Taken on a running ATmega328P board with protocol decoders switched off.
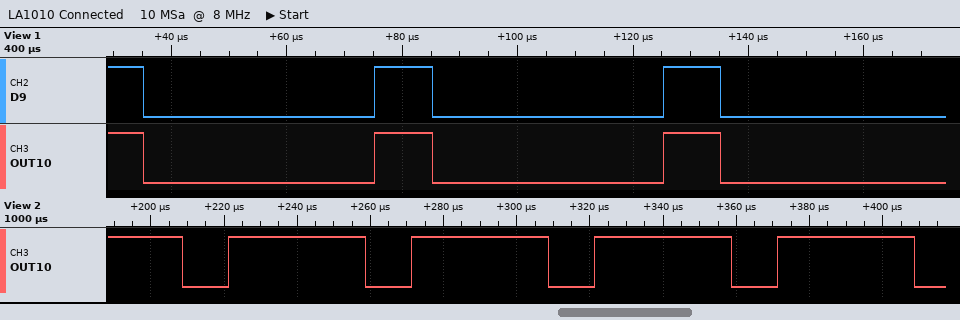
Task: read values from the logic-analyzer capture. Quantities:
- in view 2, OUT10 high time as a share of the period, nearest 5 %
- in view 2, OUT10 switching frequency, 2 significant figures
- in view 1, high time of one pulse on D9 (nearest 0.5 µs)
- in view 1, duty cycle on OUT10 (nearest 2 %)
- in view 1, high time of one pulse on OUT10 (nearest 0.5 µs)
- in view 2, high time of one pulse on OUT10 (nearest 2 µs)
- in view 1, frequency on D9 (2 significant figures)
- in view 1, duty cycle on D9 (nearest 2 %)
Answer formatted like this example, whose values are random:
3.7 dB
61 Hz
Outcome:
75 %
20 kHz
10.0 µs
20 %
10.0 µs
38 µs
20 kHz
20 %
